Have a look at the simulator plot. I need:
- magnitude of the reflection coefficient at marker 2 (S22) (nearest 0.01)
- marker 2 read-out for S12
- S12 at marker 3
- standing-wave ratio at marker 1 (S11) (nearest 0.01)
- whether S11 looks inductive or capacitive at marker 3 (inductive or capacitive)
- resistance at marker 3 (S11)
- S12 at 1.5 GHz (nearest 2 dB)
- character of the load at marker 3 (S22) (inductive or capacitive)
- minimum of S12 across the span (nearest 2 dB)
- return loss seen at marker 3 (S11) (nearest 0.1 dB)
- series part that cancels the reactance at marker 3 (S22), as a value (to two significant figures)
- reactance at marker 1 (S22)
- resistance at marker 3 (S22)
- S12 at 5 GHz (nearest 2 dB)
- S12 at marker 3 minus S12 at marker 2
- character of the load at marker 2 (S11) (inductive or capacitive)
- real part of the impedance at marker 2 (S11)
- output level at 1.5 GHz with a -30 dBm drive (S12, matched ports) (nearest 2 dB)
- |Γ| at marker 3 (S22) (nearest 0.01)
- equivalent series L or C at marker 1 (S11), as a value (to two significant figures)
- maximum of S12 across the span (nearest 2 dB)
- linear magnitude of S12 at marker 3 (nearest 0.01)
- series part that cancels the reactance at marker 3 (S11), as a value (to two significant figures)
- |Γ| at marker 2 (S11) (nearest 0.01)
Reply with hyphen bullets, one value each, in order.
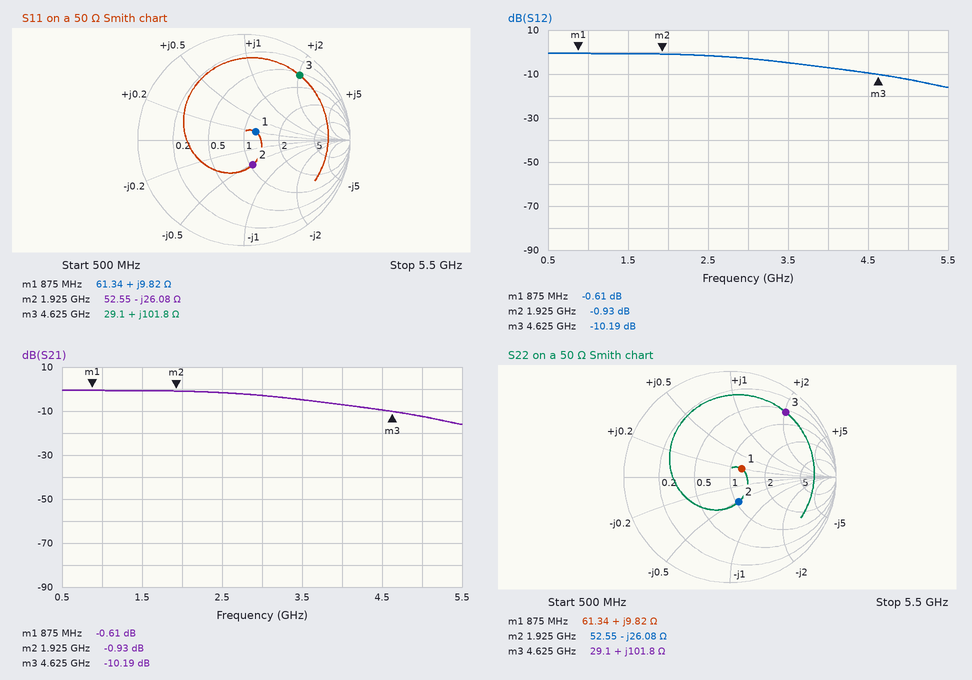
- 0.25
- -0.93 dB
- -10.19 dB
- 1.31
- inductive
- 29.1 Ω
- 0 dB
- inductive
- -16 dB
- 1.9 dB
- 340 fF
- +9.82 Ω
- 29.1 Ω
- -12 dB
- -9.26 dB
- capacitive
- 52.55 Ω
- -30 dBm
- 0.81
- 1.8 nH
- 0 dB
- 0.31
- 340 fF
- 0.25
